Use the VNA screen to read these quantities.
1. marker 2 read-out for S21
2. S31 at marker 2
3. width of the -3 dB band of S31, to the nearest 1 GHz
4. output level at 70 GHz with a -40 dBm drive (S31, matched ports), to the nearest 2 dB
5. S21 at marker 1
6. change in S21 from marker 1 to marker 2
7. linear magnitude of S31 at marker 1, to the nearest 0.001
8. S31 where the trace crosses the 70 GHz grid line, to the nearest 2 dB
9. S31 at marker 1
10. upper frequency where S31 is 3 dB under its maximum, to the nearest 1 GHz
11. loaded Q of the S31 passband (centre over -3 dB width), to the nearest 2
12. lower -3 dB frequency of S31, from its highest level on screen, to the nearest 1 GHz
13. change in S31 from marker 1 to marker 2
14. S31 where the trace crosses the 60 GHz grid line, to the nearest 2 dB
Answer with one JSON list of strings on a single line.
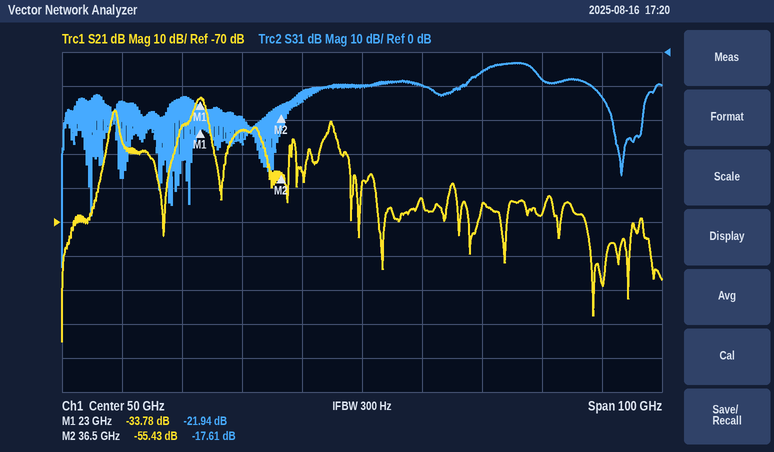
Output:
["-55.43 dB", "-17.61 dB", "9 GHz", "-46 dBm", "-33.78 dB", "-21.65 dB", "0.080", "-6 dB", "-21.94 dB", "79 GHz", "8", "70 GHz", "4.33 dB", "-10 dB"]
